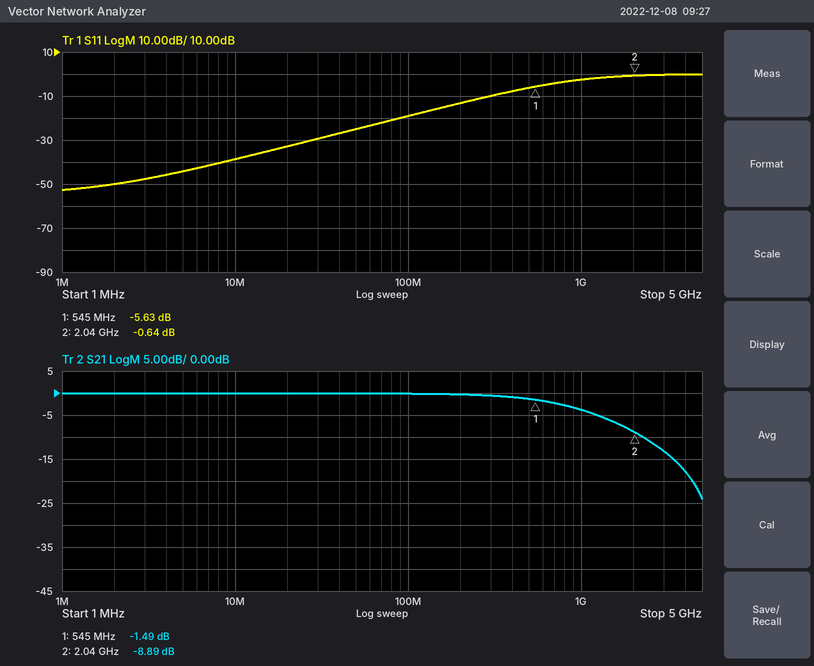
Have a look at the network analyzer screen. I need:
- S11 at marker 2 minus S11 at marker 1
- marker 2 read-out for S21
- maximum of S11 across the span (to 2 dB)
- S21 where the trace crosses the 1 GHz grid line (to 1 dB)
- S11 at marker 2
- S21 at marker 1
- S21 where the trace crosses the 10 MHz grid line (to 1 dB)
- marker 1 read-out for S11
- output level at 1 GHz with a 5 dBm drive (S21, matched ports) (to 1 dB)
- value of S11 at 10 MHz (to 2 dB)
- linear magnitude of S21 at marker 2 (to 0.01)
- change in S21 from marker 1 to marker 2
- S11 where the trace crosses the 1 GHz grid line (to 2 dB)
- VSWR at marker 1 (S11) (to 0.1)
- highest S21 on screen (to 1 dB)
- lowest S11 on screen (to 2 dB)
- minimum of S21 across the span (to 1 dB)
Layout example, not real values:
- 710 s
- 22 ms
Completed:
- 4.99 dB
- -8.89 dB
- 0 dB
- -4 dB
- -0.64 dB
- -1.49 dB
- 0 dB
- -5.63 dB
- 1 dBm
- -38 dB
- 0.36
- -7.40 dB
- -2 dB
- 3.2
- 0 dB
- -52 dB
- -24 dB
